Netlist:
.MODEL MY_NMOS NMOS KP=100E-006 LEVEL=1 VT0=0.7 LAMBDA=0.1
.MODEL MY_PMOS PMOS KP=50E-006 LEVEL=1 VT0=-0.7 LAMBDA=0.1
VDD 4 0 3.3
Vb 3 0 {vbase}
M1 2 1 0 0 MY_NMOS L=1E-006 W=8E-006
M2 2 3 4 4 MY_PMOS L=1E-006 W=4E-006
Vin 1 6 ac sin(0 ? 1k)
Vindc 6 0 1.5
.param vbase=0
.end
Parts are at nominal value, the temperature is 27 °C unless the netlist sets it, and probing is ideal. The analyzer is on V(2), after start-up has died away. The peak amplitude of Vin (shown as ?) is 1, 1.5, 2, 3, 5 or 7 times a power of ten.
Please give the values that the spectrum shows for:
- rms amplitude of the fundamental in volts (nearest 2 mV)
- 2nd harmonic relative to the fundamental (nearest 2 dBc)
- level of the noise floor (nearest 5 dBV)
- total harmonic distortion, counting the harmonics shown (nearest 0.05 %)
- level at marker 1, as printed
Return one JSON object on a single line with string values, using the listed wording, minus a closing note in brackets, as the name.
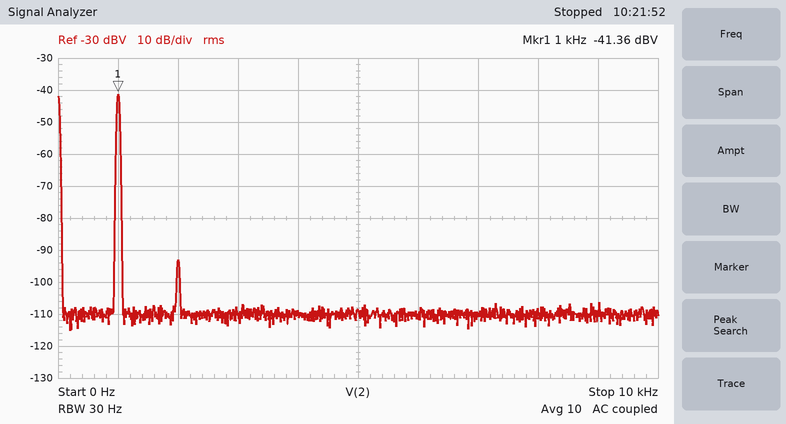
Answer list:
{"rms amplitude of the fundamental in volts": "8 mV", "2nd harmonic relative to the fundamental": "-52 dBc", "level of the noise floor": "-110 dBV", "total harmonic distortion, counting the harmonics shown": "0.25 %", "level at marker 1, as printed": "-41.36 dBV"}
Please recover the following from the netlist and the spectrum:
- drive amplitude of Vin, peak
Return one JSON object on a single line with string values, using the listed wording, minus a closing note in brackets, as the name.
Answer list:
{"drive amplitude of Vin, peak": "7 mV"}
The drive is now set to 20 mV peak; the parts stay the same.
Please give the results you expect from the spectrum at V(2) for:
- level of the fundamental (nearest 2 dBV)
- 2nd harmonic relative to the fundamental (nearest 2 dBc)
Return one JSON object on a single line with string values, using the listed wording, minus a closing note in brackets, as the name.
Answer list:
{"level of the fundamental": "-32 dBV", "2nd harmonic relative to the fundamental": "-42 dBc"}
